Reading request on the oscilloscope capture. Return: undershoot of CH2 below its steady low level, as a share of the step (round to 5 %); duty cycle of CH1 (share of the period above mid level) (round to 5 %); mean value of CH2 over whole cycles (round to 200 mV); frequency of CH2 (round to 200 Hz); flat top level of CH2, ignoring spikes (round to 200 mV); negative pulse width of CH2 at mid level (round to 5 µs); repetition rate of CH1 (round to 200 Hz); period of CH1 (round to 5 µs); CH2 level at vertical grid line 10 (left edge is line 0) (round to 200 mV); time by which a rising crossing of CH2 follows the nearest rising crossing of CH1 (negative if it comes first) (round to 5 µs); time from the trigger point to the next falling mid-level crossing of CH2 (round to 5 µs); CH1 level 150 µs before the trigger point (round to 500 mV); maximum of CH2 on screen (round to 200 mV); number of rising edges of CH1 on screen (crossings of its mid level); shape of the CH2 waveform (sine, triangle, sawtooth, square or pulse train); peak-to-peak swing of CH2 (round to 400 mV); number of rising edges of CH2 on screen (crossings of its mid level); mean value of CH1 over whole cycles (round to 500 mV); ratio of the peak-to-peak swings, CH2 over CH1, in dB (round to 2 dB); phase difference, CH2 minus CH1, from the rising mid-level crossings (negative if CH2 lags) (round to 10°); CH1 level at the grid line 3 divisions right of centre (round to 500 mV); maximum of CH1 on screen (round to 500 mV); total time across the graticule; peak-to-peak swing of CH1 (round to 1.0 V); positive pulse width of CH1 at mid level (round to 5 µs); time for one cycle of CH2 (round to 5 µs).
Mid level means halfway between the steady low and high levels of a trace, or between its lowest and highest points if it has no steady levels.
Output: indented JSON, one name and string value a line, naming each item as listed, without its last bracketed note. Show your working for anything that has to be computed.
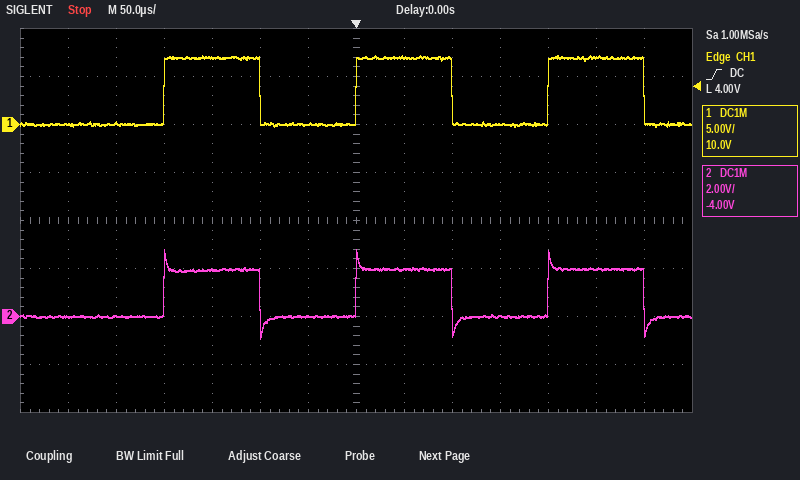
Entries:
{
  "undershoot of CH2 below its steady low level, as a share of the step": "45 %",
  "duty cycle of CH1 (share of the period above mid level)": "100 µs / 200 µs ≈ 50 %",
  "mean value of CH2 over whole cycles": "0.0 V + 0.5 × (2.0 V − (0.0 V)) ≈ 1.0 V",
  "frequency of CH2": "1 / 200 µs ≈ 5.0 kHz",
  "flat top level of CH2, ignoring spikes": "2.0 V",
  "negative pulse width of CH2 at mid level": "100 µs",
  "repetition rate of CH1": "1 / 200 µs ≈ 5.0 kHz",
  "period of CH1": "200 µs",
  "CH2 level at vertical grid line 10 (left edge is line 0)": "0.0 V",
  "time by which a rising crossing of CH2 follows the nearest rising crossing of CH1 (negative if it comes first)": "0 µs",
  "time from the trigger point to the next falling mid-level crossing of CH2": "100 µs",
  "CH1 level 150 µs before the trigger point": "7.0 V",
  "maximum of CH2 on screen": "2.8 V",
  "number of rising edges of CH1 on screen": "3",
  "shape of the CH2 waveform": "square",
  "peak-to-peak swing of CH2": "3.6 V",
  "number of rising edges of CH2 on screen": "3",
  "mean value of CH1 over whole cycles": "0.0 V + 0.5 × (7.0 V − (0.0 V)) ≈ 3.5 V",
  "ratio of the peak-to-peak swings, CH2 over CH1, in dB": "20 log10(3.6 V / 7.0 V) ≈ -6 dB",
  "phase difference, CH2 minus CH1, from the rising mid-level crossings (negative if CH2 lags)": "−360° × (0 µs) / 200 µs ≈ 0°",
  "CH1 level at the grid line 3 divisions right of centre": "0.0 V",
  "maximum of CH1 on screen": "7.0 V",
  "total time across the graticule": "700 µs",
  "peak-to-peak swing of CH1": "7.0 V",
  "positive pulse width of CH1 at mid level": "100 µs",
  "time for one cycle of CH2": "200 µs"
}
